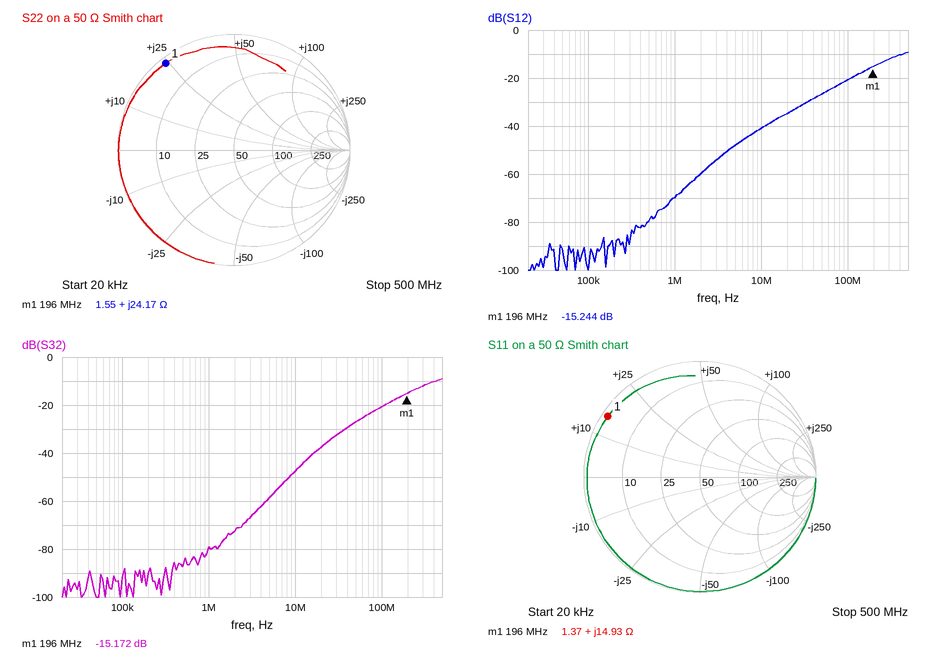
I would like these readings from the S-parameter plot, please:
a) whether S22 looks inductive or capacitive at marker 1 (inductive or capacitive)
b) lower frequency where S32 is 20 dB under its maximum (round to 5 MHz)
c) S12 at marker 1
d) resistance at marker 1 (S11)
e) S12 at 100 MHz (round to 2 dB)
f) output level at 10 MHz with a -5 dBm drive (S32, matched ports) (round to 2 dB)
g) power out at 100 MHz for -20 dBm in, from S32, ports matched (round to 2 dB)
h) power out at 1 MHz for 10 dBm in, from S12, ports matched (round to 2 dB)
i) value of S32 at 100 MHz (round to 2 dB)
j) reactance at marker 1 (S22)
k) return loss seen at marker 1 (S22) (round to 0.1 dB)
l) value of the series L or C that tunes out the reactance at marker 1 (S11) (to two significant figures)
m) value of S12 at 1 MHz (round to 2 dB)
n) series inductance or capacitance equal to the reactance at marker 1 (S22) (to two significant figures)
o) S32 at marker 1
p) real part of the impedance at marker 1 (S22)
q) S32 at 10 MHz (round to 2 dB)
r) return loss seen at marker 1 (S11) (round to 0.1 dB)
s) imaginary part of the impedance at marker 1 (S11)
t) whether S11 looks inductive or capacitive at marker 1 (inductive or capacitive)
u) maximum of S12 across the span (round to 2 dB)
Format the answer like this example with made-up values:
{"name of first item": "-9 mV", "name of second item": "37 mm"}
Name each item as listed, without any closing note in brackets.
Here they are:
{"whether S22 looks inductive or capacitive at marker 1": "inductive", "lower frequency where S32 is 20 dB under its maximum": "40 MHz", "S12 at marker 1": "-15.244 dB", "resistance at marker 1": "1.37 Ω", "S12 at 100 MHz": "-20 dB", "output level at 10 MHz with a -5 dBm drive (S32, matched ports)": "-52 dBm", "power out at 100 MHz for -20 dBm in, from S32, ports matched": "-40 dBm", "power out at 1 MHz for 10 dBm in, from S12, ports matched": "-60 dBm", "value of S32 at 100 MHz": "-20 dB", "reactance at marker 1": "+24.17 Ω", "return loss seen at marker 1 (S22)": "0.4 dB", "value of the series L or C that tunes out the reactance at marker 1 (S11)": "54 pF", "value of S12 at 1 MHz": "-70 dB", "series inductance or capacitance equal to the reactance at marker 1 (S22)": "20 nH", "S32 at marker 1": "-15.172 dB", "real part of the impedance at marker 1": "1.55 Ω", "S32 at 10 MHz": "-48 dB", "return loss seen at marker 1 (S11)": "0.4 dB", "imaginary part of the impedance at marker 1": "+14.93 Ω", "whether S11 looks inductive or capacitive at marker 1": "inductive", "maximum of S12 across the span": "-10 dB"}
